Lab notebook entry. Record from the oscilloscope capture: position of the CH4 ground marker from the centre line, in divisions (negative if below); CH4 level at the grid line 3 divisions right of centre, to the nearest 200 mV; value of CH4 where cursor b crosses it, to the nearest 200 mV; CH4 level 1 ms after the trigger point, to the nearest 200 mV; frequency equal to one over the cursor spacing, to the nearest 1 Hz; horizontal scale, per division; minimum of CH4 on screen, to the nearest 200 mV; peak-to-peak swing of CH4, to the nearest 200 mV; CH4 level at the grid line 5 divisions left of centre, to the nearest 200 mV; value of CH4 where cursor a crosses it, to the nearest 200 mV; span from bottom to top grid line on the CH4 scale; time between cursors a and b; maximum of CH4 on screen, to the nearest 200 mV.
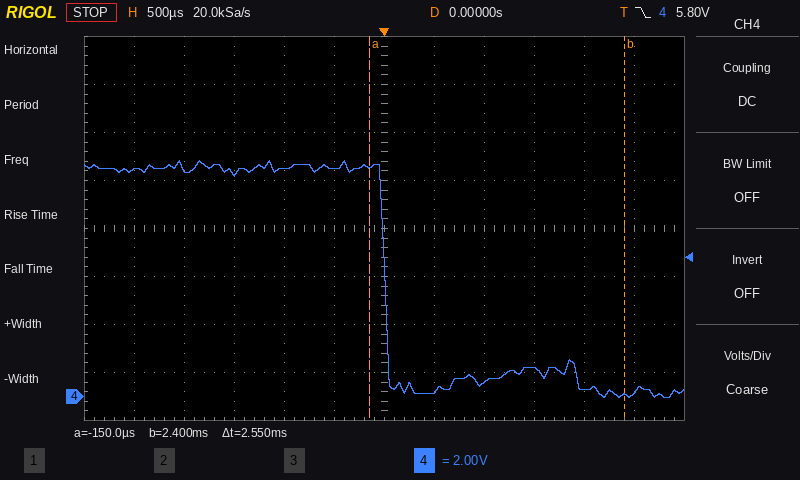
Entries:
-3.5 div
1.2 V
0.0 V
600 mV
392 Hz
500 µs
0.0 V
9.8 V
9.4 V
9.6 V
16 V
2.55 ms
9.8 V
